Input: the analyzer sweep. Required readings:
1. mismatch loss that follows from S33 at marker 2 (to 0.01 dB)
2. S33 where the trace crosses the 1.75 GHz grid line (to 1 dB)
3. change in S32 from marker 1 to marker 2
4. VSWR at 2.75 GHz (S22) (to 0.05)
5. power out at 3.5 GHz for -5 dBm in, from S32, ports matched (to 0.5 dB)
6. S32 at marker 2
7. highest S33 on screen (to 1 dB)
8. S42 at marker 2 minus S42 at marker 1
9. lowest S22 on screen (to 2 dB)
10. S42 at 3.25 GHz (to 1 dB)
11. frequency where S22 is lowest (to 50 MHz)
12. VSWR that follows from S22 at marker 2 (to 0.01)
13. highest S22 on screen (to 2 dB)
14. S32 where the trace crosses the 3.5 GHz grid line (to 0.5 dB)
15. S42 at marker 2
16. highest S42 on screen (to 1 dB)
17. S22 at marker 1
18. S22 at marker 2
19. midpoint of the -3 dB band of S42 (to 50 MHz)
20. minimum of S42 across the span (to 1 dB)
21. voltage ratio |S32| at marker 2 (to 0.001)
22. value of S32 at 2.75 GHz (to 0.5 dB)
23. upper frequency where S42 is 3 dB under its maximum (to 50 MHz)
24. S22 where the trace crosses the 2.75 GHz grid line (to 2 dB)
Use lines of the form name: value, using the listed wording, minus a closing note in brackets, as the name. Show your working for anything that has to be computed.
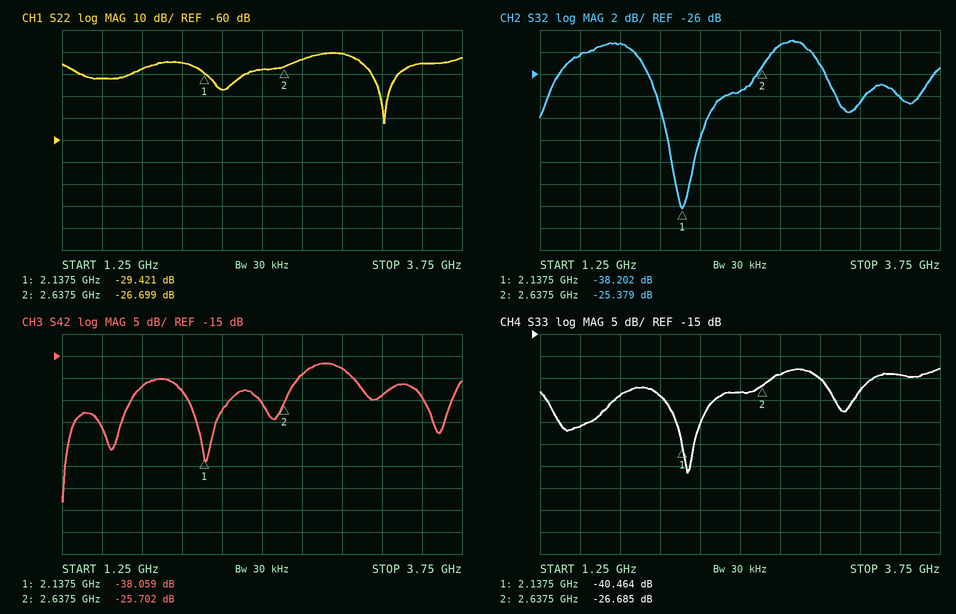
mismatch loss that follows from S33 at marker 2: −10 log10(1 − 10^(-26.685/10)) ≈ 0.01 dB
S33 where the trace crosses the 1.75 GHz grid line: -29 dB
change in S32 from marker 1 to marker 2: -25.379 − (-38.202) = 12.823 dB
VSWR at 2.75 GHz (S22): |Γ| = 10^(-24/20) = 0.0631; VSWR = (1 + 0.0631)/(1 − 0.0631) ≈ 1.13, so 1.15 to the nearest 0.05
power out at 3.5 GHz for -5 dBm in, from S32, ports matched: -5 dBm + (-28.0 dB) = -33.0 dBm
S32 at marker 2: -25.379 dB
highest S33 on screen: -23 dB
S42 at marker 2 minus S42 at marker 1: -25.702 − (-38.059) = 12.357 dB
lowest S22 on screen: -52 dB
S42 at 3.25 GHz: -24 dB
frequency where S22 is lowest: 3.25 GHz
VSWR that follows from S22 at marker 2: (1 + 0.0462)/(1 − 0.0462) ≈ 1.10
highest S22 on screen: -20 dB
S32 where the trace crosses the 3.5 GHz grid line: -28.0 dB
S42 at marker 2: -25.702 dB
highest S42 on screen: -17 dB
S22 at marker 1: -29.421 dB
S22 at marker 2: -26.699 dB
midpoint of the -3 dB band of S42: 2.90 GHz
minimum of S42 across the span: -48 dB
voltage ratio |S32| at marker 2: 10^(-25.379/20) ≈ 0.054
value of S32 at 2.75 GHz: -23.5 dB
upper frequency where S42 is 3 dB under its maximum: 3.05 GHz
S22 where the trace crosses the 2.75 GHz grid line: -24 dB
